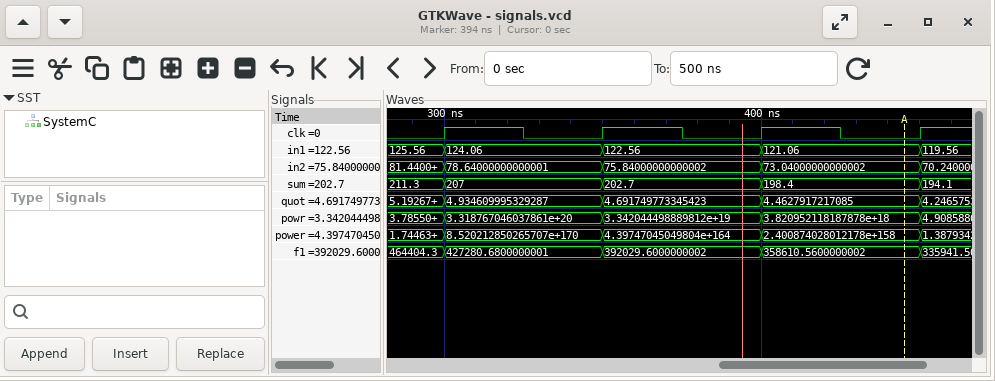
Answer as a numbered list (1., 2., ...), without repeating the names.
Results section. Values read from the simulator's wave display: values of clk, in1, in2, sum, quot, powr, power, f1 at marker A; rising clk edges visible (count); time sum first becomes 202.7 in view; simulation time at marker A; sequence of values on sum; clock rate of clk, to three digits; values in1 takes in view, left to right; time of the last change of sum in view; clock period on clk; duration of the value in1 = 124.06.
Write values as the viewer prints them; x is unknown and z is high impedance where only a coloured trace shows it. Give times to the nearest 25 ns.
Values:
1. clk=0, in1=121.06, in2=73.04000000000002, sum=198.4, quot=4.4627917217085, powr=3.820952118187878e+18, power=2.400874028012178e+158, f1=358610.5600000002
2. 4
3. 350 ns
4. 450 ns
5. 211.3, 207, 202.7, 198.4, 194.1
6. 20.0 MHz
7. 125.56, 124.06, 122.56, 121.06, 119.56
8. 450 ns
9. 50 ns
10. 50 ns
